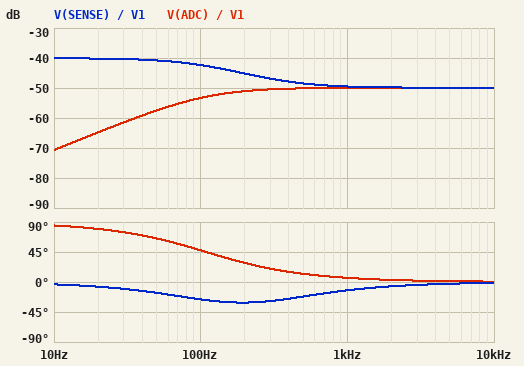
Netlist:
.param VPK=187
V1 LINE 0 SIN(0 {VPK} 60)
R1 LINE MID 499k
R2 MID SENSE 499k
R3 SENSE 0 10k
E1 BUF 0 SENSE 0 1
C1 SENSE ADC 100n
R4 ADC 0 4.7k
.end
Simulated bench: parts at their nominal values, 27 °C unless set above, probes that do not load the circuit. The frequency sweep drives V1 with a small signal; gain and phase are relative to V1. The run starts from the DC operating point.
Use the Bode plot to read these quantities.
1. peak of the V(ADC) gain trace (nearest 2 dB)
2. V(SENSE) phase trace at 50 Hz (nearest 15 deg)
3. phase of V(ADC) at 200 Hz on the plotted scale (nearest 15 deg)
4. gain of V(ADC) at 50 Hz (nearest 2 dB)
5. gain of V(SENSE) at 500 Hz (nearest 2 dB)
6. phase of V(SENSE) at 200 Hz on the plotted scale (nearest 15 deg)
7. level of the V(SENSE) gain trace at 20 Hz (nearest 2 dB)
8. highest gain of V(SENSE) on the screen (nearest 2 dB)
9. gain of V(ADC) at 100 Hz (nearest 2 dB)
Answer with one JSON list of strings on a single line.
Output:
["-50 dB", "-15 deg", "30 deg", "-58 dB", "-48 dB", "-30 deg", "-40 dB", "-40 dB", "-54 dB"]
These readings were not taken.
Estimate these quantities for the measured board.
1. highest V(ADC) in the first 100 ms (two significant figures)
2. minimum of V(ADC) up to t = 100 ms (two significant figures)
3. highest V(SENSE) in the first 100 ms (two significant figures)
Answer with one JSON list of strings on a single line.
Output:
["290 mV", "-290 mV", "1.7 V"]
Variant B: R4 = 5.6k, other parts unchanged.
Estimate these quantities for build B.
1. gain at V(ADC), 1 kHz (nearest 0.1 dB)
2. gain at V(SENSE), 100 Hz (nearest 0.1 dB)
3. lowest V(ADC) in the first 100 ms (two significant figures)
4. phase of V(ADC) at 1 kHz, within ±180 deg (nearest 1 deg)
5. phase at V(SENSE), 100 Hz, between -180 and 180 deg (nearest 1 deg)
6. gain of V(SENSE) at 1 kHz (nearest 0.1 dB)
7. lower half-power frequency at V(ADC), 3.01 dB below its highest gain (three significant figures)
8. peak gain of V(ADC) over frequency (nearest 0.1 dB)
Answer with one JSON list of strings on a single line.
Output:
["-49.0 dB", "-42.5 dB", "-340 mV", "6 deg", "-25 deg", "-48.6 dB", "103 Hz", "-48.9 dB"]
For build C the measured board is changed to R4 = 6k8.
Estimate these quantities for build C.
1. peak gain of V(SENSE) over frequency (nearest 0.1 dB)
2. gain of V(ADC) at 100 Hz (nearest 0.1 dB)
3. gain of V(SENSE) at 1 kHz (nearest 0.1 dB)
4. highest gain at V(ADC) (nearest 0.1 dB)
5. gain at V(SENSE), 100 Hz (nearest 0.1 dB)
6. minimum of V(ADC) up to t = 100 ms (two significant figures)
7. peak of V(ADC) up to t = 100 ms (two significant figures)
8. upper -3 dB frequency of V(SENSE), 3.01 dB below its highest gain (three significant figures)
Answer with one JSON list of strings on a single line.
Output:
["-40.1 dB", "-50.7 dB", "-47.7 dB", "-47.9 dB", "-42.6 dB", "-400 mV", "400 mV", "117 Hz"]
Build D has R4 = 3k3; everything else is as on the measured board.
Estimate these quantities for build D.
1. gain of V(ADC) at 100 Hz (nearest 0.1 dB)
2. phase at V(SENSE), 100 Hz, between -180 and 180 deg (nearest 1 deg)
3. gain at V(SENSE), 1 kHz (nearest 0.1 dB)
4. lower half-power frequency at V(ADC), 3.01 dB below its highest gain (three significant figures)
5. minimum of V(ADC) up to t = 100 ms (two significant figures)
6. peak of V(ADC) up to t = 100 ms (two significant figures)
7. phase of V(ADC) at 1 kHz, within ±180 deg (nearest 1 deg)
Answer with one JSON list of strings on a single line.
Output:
["-56.0 dB", "-28 deg", "-51.3 dB", "121 Hz", "-210 mV", "210 mV", "7 deg"]
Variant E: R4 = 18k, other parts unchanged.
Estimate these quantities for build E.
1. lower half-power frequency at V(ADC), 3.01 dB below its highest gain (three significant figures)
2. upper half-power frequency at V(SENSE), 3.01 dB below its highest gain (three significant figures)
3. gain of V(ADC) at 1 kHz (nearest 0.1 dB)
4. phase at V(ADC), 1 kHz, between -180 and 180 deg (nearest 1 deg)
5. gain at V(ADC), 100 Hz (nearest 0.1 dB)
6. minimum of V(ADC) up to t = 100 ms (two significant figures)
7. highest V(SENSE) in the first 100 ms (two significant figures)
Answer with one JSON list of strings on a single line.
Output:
["57.0 Hz", "139 Hz", "-43.9 dB", "3 deg", "-45.1 dB", "-880 mV", "1.6 V"]
